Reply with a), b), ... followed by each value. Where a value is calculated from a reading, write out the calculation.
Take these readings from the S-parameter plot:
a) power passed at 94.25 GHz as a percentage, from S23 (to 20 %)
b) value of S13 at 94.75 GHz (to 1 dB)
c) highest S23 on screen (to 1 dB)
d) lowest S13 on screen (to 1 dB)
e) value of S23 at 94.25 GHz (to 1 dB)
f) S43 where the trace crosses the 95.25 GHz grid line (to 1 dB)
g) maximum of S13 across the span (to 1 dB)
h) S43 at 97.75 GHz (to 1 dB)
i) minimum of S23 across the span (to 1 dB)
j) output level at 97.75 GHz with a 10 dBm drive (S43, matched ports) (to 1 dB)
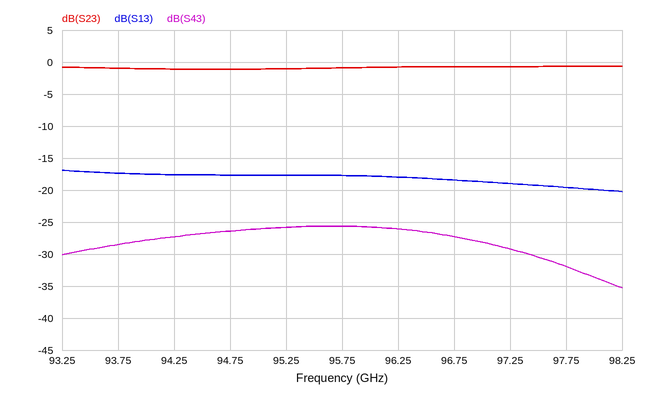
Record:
a) 10^(-1/10) ≈ 79.4 %, so 80 % to the nearest 20 %
b) -18 dB
c) -1 dB
d) -20 dB
e) -1 dB
f) -26 dB
g) -17 dB
h) -32 dB
i) -1 dB
j) 10 dBm + (-32 dB) = -22 dBm
